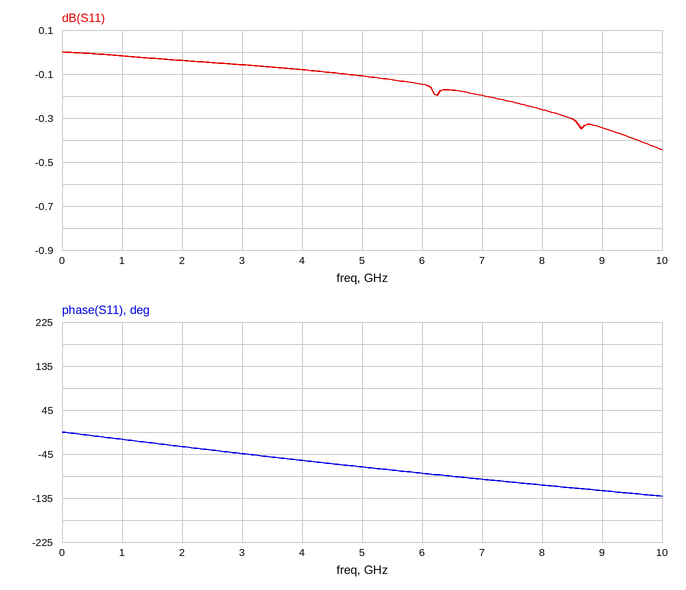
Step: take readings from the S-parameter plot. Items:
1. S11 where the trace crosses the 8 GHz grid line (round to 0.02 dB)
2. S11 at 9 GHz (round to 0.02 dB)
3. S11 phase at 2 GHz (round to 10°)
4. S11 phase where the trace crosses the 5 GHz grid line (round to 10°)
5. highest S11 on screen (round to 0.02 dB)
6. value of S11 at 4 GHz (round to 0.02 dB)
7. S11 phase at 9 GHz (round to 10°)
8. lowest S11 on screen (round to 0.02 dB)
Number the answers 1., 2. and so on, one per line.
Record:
1. -0.26 dB
2. -0.34 dB
3. -30°
4. -70°
5. 0.00 dB
6. -0.08 dB
7. -120°
8. -0.44 dB
